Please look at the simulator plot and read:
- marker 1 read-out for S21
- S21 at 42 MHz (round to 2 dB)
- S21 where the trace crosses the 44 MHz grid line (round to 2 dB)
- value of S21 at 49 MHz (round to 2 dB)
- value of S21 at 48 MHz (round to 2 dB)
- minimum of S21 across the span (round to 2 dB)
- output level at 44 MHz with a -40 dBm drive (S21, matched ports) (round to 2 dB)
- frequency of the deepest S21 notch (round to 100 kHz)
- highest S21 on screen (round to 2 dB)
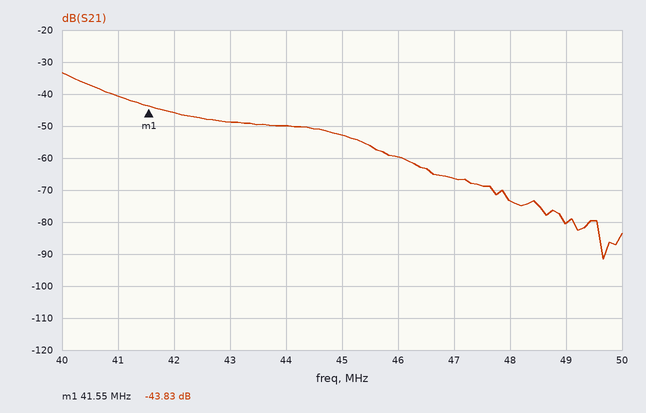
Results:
-43.83 dB
-46 dB
-50 dB
-80 dB
-74 dB
-92 dB
-90 dBm
49.7 MHz
-34 dB
